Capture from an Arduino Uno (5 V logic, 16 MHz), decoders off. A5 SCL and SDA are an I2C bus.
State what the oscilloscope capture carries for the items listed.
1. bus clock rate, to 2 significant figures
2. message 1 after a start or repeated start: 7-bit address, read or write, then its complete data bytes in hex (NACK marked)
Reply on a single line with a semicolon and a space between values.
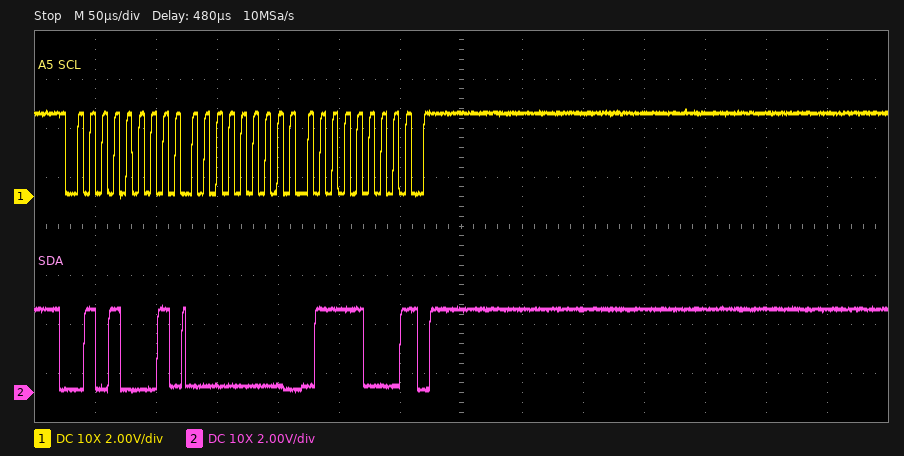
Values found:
100 kHz; 0x28 read: 00 78 NACK
